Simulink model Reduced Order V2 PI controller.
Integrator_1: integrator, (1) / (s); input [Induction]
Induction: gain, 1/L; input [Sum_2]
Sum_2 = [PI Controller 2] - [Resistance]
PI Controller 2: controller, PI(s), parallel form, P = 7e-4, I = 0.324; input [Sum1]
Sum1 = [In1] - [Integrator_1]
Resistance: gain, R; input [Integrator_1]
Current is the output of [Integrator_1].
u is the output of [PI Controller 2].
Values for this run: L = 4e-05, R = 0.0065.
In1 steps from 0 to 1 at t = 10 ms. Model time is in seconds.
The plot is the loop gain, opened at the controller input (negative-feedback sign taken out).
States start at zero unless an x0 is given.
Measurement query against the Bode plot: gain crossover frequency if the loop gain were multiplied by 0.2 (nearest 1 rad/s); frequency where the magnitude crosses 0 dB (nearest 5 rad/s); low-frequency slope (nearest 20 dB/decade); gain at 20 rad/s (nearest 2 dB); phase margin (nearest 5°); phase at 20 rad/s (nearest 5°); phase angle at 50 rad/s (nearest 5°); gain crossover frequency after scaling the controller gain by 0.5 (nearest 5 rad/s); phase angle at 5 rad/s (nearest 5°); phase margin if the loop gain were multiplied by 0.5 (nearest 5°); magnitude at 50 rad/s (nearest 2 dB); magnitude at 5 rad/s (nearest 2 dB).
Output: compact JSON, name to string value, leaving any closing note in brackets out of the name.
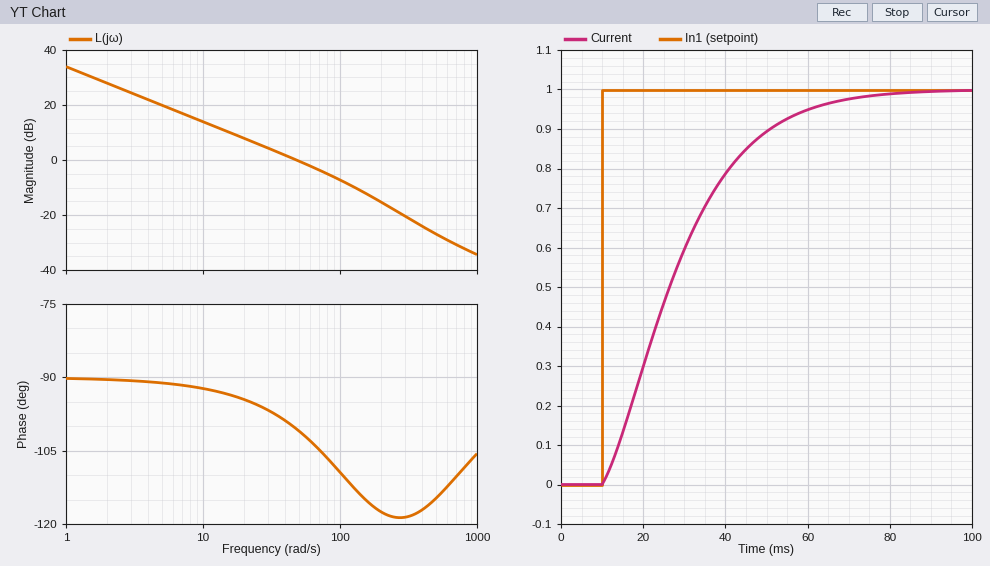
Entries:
{"gain crossover frequency if the loop gain were multiplied by 0.2": "10 rad/s", "frequency where the magnitude crosses 0 dB": "50 rad/s", "low-frequency slope": "-20 dB/decade", "gain at 20 rad/s": "8 dB", "phase margin": "80°", "phase at 20 rad/s": "-95°", "phase angle at 50 rad/s": "-100°", "gain crossover frequency after scaling the controller gain by 0.5": "25 rad/s", "phase angle at 5 rad/s": "-90°", "phase margin if the loop gain were multiplied by 0.5": "85°", "magnitude at 50 rad/s": "0 dB", "magnitude at 5 rad/s": "20 dB"}
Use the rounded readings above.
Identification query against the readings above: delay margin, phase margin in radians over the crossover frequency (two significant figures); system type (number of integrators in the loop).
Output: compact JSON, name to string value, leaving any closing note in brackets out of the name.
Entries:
{"delay margin, phase margin in radians over the crossover frequency": "0.028 s", "system type": "1"}
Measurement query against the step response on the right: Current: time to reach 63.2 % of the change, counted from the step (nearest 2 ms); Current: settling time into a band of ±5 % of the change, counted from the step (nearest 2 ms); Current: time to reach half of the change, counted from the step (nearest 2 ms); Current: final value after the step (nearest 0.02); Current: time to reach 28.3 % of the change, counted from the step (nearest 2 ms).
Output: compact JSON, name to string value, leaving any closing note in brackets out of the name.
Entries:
{"Current: time to reach 63.2 % of the change, counted from the step": "22 ms", "Current: settling time into a band of ±5 % of the change, counted from the step": "50 ms", "Current: time to reach half of the change, counted from the step": "16 ms", "Current: final value after the step": "1.00", "Current: time to reach 28.3 % of the change, counted from the step": "10 ms"}
